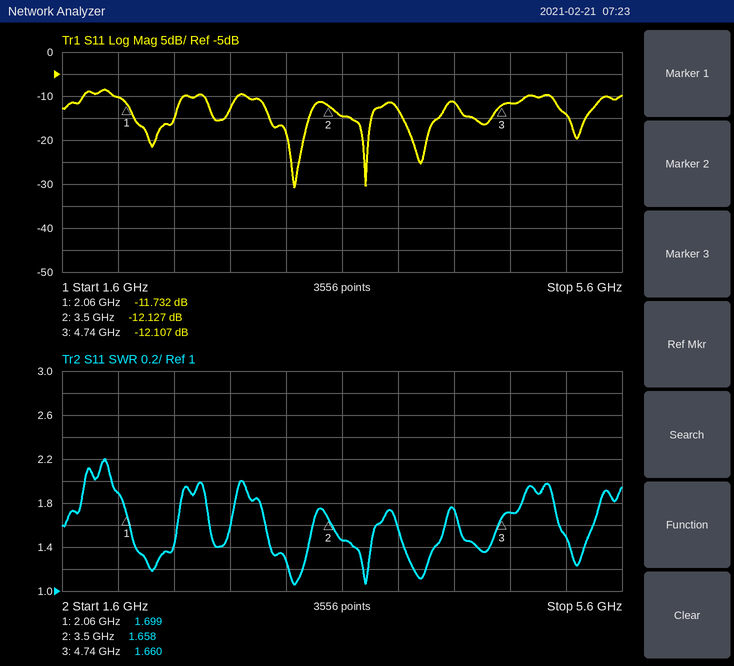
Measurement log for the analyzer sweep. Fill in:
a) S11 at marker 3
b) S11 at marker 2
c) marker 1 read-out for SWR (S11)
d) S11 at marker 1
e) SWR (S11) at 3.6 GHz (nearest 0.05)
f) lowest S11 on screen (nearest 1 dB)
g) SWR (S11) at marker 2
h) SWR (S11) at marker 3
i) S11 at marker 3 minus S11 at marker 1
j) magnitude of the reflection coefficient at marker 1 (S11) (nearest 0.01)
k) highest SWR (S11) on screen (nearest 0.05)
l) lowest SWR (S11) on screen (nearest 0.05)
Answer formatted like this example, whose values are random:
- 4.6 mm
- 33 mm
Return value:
- -12.107 dB
- -12.127 dB
- 1.699
- -11.732 dB
- 1.45
- -31 dB
- 1.658
- 1.660
- -0.375 dB
- 0.26
- 2.20
- 1.05
